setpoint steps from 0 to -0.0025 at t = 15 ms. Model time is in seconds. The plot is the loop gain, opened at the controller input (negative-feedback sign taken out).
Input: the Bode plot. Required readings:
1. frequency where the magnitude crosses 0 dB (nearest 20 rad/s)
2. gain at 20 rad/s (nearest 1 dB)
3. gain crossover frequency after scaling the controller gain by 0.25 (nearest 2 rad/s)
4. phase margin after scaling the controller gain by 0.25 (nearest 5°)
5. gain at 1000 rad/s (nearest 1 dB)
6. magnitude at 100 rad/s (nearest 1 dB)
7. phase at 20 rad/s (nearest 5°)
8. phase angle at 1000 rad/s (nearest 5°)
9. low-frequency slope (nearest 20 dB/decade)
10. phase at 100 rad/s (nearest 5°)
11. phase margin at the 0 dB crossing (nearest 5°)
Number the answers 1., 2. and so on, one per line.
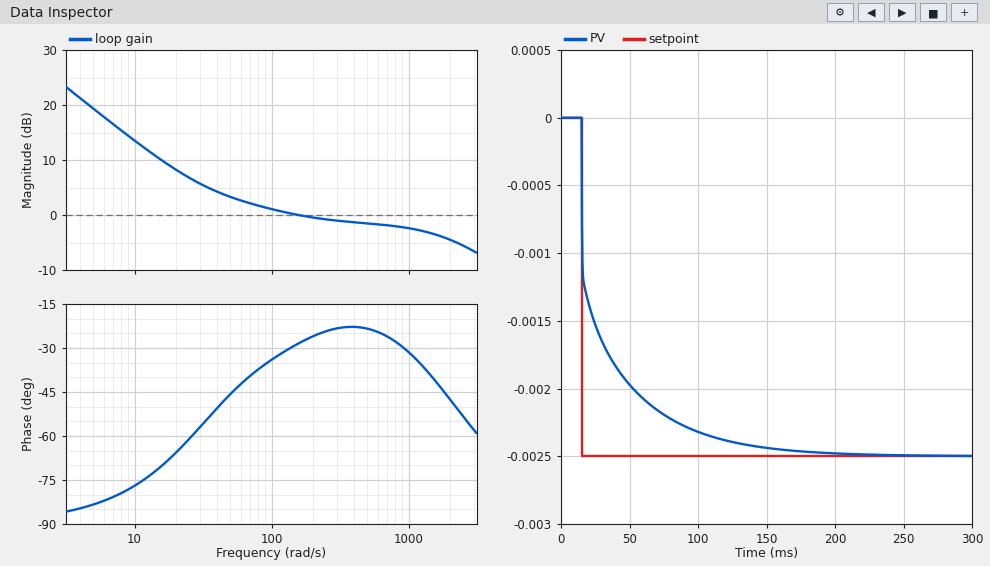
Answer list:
1. 160 rad/s
2. 8 dB
3. 12 rad/s
4. 105°
5. -2 dB
6. 1 dB
7. -65°
8. -30°
9. -20 dB/decade
10. -35°
11. 150°
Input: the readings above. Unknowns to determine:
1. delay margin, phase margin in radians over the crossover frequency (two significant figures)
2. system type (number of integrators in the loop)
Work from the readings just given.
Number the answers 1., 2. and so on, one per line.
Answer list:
1. 0.016 s
2. 1
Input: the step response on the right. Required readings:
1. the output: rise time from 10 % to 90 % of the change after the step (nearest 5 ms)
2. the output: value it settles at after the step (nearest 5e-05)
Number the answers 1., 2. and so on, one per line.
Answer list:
1. 70 ms
2. -0.00250
